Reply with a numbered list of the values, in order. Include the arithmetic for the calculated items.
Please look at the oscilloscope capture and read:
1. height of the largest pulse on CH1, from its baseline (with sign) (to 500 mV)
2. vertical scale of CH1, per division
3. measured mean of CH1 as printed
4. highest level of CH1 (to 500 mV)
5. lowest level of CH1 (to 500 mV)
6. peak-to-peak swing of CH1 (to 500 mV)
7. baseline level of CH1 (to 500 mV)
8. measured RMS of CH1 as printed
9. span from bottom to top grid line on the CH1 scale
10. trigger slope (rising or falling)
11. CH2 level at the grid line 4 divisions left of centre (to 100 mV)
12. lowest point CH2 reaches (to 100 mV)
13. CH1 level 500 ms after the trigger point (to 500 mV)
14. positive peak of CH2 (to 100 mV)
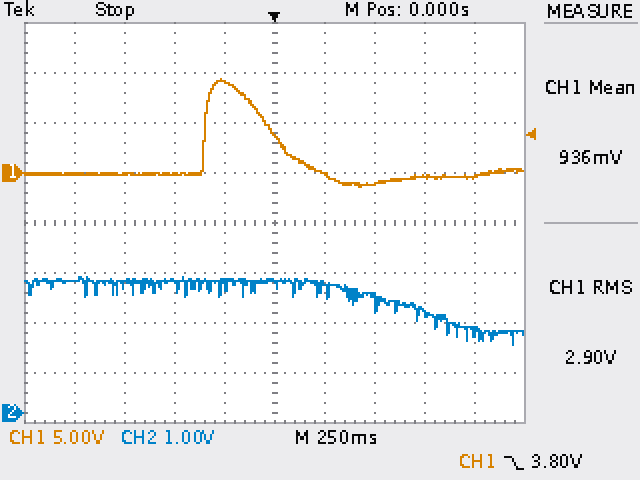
1. 9.5 V − (0.0 V) = +9.5 V
2. 5 V
3. 936 mV
4. 9.5 V
5. -1.5 V
6. 9.5 V − (-1.5 V) = 11.0 V
7. 0.0 V
8. 2.90 V
9. 40 V
10. falling
11. 2.6 V
12. 1.4 V
13. -1.0 V
14. 2.7 V
